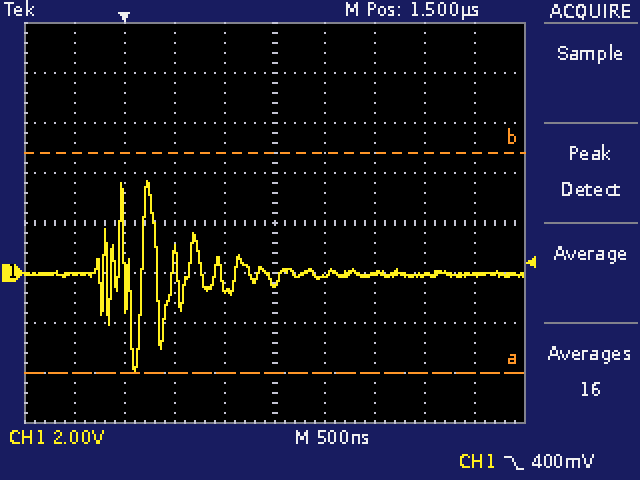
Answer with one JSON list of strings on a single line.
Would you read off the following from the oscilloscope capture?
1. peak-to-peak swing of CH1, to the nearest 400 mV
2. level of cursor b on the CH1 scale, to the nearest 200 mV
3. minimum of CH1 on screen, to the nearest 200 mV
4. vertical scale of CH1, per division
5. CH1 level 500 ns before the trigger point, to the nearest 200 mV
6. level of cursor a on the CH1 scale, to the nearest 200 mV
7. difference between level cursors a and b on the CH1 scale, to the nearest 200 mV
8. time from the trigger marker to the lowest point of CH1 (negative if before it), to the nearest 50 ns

["7.6 V", "4.8 V", "-4.0 V", "2 V", "0.0 V", "-4.0 V", "8.8 V", "+100 ns"]
